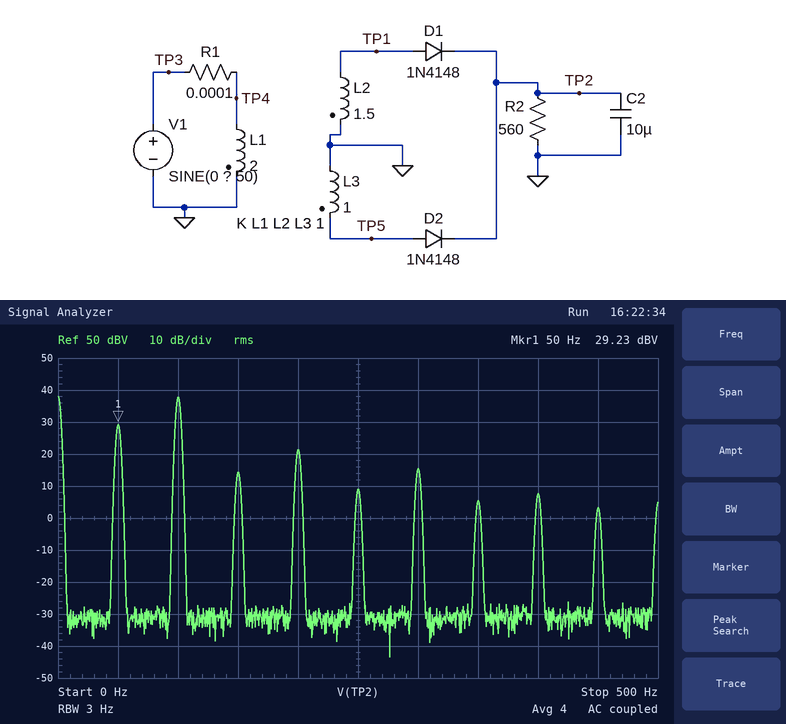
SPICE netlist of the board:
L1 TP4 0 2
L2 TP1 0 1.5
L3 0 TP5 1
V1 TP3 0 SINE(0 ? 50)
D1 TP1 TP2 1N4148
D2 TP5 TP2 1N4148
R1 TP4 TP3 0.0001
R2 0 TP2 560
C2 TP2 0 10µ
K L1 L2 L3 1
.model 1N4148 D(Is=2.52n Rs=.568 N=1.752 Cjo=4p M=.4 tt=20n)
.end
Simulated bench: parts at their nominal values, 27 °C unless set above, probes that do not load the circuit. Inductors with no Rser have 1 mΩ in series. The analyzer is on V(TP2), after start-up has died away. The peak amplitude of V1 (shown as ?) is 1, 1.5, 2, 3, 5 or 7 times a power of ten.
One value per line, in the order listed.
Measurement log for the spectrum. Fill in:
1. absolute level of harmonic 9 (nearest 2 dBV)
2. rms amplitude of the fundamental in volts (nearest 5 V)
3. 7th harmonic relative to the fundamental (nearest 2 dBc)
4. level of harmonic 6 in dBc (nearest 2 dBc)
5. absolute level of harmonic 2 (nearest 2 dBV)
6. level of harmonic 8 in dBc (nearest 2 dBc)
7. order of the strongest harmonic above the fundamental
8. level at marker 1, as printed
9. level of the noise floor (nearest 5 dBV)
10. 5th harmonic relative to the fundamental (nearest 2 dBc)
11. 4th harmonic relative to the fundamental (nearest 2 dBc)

4 dBV
30 V
-24 dBc
-14 dBc
38 dBV
-22 dBc
2
29.23 dBV
-30 dBV
-20 dBc
-8 dBc
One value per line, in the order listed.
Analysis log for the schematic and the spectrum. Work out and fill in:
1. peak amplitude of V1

500 V
